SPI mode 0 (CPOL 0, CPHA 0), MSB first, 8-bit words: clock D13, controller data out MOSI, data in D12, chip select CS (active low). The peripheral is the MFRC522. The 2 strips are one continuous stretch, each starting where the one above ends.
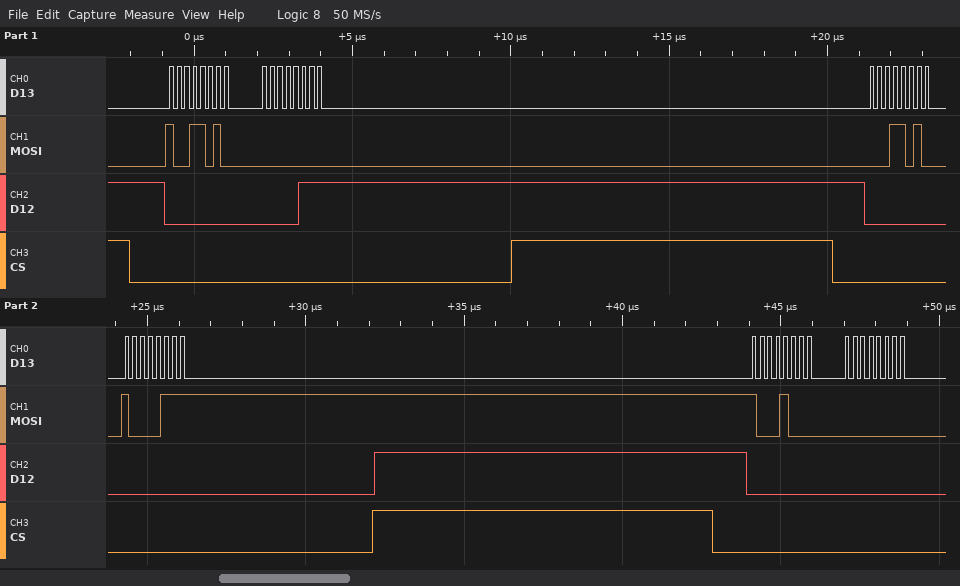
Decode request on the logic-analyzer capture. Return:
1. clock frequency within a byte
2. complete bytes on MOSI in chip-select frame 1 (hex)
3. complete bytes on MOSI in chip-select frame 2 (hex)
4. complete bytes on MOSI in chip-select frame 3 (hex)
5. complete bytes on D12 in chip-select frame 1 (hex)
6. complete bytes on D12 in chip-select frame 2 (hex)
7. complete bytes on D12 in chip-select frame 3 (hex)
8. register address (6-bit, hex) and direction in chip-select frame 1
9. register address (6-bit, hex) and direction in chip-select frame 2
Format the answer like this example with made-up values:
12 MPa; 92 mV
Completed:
4 MHz; 0x9A 0x00; 0x1A 0x87; 0x88 0x00; 0x00 0x07; 0x00 0x00; 0x00 0x00; 0x0D read; 0x0D write
